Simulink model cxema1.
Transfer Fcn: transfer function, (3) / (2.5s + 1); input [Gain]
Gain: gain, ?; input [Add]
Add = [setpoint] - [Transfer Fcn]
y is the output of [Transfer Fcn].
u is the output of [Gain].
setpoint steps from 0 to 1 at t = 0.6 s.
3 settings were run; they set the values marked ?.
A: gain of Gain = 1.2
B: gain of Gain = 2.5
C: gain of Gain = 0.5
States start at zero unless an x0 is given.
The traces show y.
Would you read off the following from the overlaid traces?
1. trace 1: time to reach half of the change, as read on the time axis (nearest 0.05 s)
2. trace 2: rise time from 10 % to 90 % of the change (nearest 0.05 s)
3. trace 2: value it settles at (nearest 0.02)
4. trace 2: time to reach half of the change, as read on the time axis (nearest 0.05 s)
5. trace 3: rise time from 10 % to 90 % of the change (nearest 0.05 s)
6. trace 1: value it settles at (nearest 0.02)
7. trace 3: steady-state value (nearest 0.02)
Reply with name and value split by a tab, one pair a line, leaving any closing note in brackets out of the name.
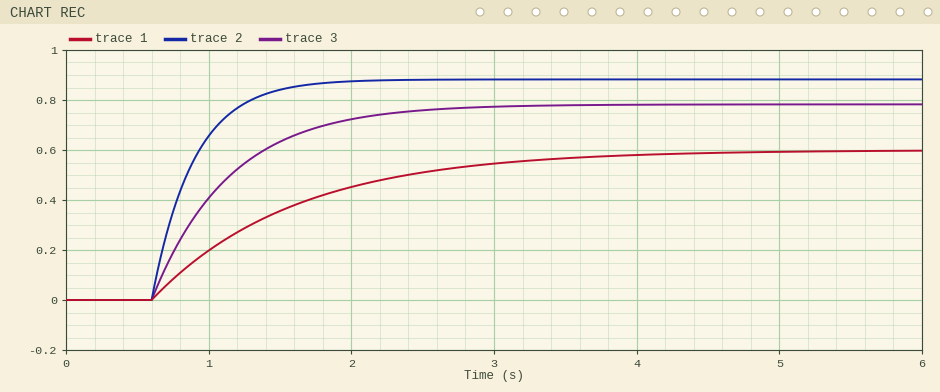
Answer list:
trace 1: time to reach half of the change, as read on the time axis	1.30 s
trace 2: rise time from 10 % to 90 % of the change	0.65 s
trace 2: value it settles at	0.88
trace 2: time to reach half of the change, as read on the time axis	0.80 s
trace 3: rise time from 10 % to 90 % of the change	1.20 s
trace 1: value it settles at	0.60
trace 3: steady-state value	0.78
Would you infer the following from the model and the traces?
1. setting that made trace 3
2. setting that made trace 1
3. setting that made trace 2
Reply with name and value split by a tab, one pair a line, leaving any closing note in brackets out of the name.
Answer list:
setting that made trace 3	A
setting that made trace 1	C
setting that made trace 2	B
